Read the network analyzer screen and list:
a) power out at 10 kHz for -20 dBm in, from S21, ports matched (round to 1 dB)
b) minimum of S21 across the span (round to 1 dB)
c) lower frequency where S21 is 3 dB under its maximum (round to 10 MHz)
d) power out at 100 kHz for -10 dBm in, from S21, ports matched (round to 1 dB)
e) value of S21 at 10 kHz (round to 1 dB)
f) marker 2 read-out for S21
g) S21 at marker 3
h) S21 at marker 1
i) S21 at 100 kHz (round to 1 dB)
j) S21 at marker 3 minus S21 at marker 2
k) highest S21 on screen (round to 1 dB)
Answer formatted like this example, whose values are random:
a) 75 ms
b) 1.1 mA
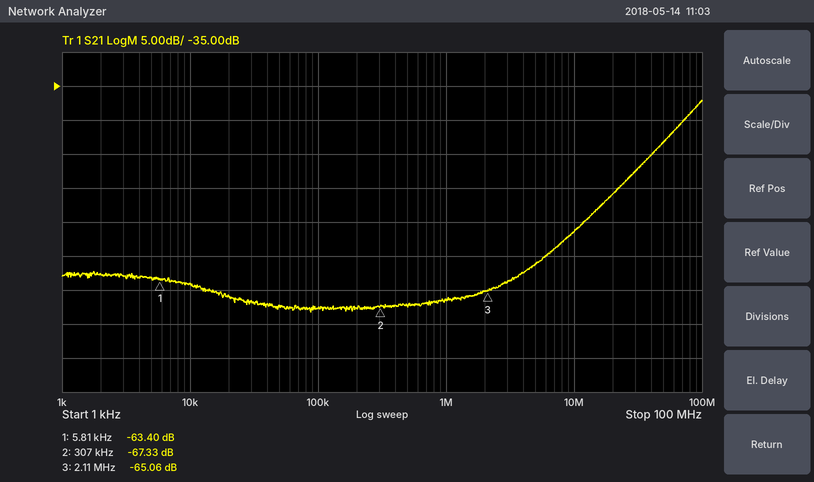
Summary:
a) -84 dBm
b) -68 dB
c) 70 MHz
d) -78 dBm
e) -64 dB
f) -67.33 dB
g) -65.06 dB
h) -63.40 dB
i) -68 dB
j) 2.27 dB
k) -37 dB
